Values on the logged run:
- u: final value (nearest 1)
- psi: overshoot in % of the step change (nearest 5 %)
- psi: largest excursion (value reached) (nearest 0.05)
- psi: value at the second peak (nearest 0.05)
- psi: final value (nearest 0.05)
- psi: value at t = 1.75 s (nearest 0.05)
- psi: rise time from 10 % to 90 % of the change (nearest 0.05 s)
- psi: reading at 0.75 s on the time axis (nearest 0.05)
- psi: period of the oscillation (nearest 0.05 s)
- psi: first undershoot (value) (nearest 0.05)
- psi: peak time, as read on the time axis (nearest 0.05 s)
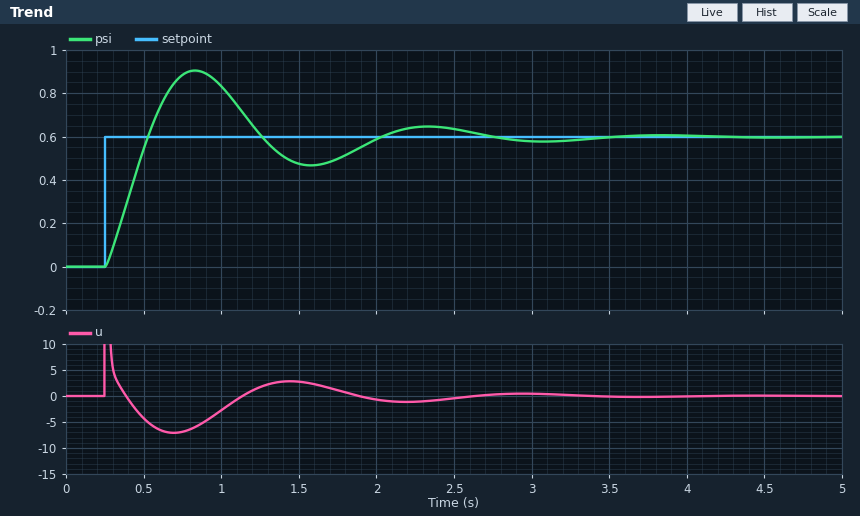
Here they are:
0
50 %
0.90
0.65
0.60
0.50
0.20 s
0.90
1.50 s
0.45
0.85 s
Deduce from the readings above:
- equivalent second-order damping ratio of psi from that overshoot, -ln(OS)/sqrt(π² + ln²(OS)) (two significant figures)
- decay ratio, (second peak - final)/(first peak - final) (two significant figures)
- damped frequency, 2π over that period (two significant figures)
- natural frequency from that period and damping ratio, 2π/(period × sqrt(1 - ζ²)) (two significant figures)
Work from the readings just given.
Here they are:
0.22
0.17
4.2 rad/s
4.3 rad/s
